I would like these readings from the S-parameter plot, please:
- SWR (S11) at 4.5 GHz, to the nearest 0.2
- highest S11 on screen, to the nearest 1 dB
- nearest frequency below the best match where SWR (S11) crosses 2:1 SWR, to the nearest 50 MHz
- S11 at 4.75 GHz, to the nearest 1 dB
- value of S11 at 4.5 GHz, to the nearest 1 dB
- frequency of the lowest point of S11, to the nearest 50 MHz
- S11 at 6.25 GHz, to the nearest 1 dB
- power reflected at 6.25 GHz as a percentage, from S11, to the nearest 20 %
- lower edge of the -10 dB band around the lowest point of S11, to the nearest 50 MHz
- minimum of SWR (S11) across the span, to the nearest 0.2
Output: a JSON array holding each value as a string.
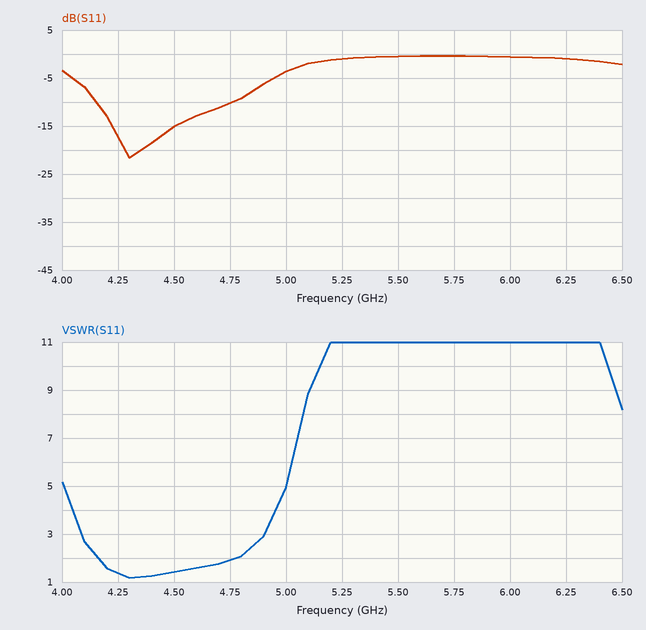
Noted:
["1.4", "0 dB", "4.15 GHz", "-10 dB", "-15 dB", "4.30 GHz", "-1 dB", "80 %", "4.15 GHz", "1.2"]
